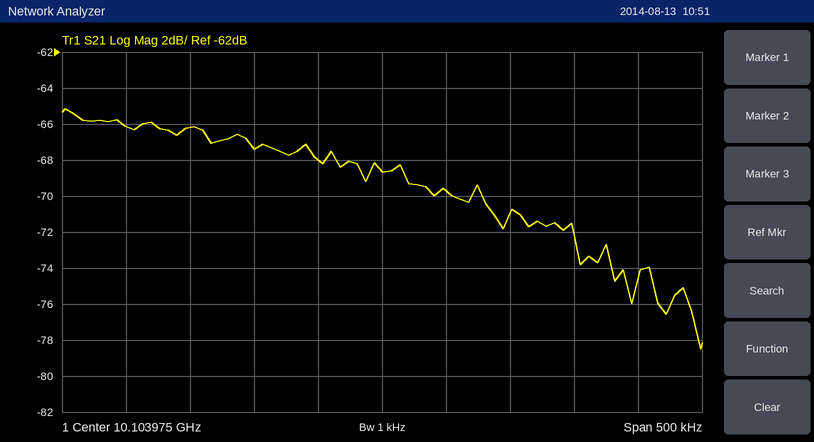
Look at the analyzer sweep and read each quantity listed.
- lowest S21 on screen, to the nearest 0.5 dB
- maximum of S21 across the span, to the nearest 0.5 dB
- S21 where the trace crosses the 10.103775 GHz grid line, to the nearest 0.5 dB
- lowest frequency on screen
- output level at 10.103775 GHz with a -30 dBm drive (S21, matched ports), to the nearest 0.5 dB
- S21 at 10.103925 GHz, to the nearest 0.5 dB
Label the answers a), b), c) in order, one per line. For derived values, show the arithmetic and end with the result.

a) -78.5 dB
b) -65.0 dB
c) -66.0 dB
d) 10.103725 GHz
e) -30 dBm + (-66.0 dB) = -96.0 dBm
f) -68.0 dB
